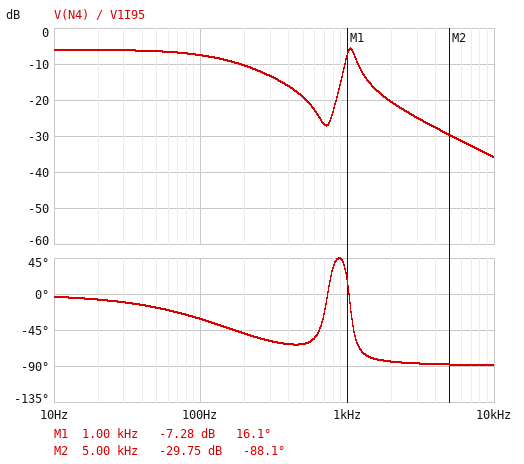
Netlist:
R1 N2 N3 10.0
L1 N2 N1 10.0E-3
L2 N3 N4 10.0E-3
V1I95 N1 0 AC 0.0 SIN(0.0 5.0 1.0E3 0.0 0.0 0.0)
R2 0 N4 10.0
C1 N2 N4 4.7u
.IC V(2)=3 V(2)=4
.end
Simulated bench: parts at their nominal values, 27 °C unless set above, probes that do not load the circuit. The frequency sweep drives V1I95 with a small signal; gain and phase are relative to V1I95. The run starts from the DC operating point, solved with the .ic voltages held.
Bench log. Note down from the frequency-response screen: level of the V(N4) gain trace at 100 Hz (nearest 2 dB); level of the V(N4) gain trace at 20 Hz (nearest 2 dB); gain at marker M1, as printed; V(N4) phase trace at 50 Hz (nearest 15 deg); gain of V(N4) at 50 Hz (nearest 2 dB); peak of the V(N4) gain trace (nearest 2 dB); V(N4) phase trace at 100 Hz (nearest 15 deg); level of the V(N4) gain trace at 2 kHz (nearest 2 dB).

-8 dB
-6 dB
-7.28 dB
-15 deg
-6 dB
-6 dB
-30 deg
-20 dB
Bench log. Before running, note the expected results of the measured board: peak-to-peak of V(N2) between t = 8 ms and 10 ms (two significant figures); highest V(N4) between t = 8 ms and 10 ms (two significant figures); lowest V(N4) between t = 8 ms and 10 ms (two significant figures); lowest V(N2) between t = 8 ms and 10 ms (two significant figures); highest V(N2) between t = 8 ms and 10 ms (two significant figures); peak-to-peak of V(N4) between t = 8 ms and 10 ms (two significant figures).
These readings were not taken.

32 V
2.2 V
-2.2 V
-16 V
16 V
4.4 V
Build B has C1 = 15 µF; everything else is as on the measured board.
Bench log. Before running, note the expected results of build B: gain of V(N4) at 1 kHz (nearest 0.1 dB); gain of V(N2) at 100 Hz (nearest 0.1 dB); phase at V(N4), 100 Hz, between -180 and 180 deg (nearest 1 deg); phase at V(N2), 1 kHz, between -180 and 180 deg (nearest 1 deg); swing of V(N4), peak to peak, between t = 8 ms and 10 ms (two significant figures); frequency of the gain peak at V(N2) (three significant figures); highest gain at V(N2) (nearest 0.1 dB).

-14.2 dB
-0.9 dB
-29 deg
-129 deg
2.0 V
571 Hz
6.2 dB
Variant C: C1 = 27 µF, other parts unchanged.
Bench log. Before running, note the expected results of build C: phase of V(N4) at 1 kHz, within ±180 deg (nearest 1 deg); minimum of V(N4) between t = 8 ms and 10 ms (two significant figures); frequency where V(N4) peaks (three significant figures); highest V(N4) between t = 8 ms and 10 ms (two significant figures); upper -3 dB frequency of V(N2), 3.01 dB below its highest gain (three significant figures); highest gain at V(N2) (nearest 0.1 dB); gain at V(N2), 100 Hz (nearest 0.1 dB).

-80 deg
-870 mV
449 Hz
880 mV
497 Hz
4.3 dB
-0.8 dB
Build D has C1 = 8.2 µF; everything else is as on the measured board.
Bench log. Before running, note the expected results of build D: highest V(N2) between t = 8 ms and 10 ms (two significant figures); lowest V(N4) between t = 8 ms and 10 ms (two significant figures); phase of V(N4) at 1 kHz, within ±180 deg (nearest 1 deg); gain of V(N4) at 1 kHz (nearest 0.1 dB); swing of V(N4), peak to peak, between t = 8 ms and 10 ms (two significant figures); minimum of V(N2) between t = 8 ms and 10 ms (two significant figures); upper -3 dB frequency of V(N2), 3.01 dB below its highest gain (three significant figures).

4.0 V
-1.3 V
-71 deg
-11.4 dB
2.7 V
-4.0 V
855 Hz
